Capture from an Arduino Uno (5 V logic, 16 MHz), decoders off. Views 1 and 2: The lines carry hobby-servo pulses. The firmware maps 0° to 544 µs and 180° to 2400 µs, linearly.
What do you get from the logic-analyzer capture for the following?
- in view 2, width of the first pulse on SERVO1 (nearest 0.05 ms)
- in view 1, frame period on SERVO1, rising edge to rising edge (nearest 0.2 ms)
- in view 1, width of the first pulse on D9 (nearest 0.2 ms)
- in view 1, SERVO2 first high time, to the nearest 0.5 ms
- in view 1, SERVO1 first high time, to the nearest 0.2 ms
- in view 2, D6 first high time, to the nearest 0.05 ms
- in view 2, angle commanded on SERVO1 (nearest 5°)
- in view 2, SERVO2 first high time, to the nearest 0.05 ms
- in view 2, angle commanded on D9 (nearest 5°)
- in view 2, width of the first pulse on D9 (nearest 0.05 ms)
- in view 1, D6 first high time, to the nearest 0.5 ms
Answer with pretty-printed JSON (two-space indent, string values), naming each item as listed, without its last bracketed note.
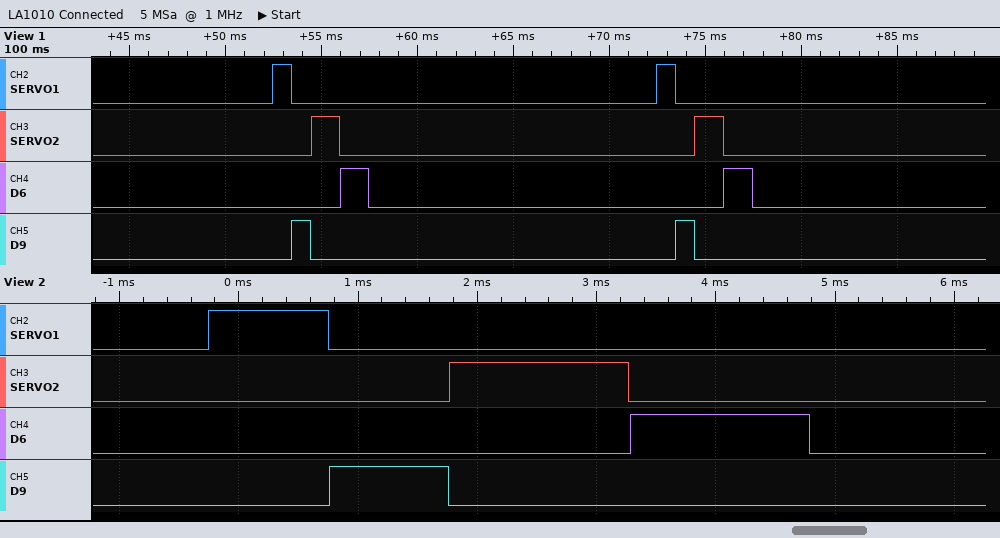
{
  "in view 2, width of the first pulse on SERVO1": "1.00 ms",
  "in view 1, frame period on SERVO1, rising edge to rising edge": "20.0 ms",
  "in view 1, width of the first pulse on D9": "1.0 ms",
  "in view 1, SERVO2 first high time, to the nearest 0.5 ms": "1.5 ms",
  "in view 1, SERVO1 first high time, to the nearest 0.2 ms": "1.0 ms",
  "in view 2, D6 first high time, to the nearest 0.05 ms": "1.50 ms",
  "in view 2, angle commanded on SERVO1": "45°",
  "in view 2, SERVO2 first high time, to the nearest 0.05 ms": "1.50 ms",
  "in view 2, angle commanded on D9": "45°",
  "in view 2, width of the first pulse on D9": "1.00 ms",
  "in view 1, D6 first high time, to the nearest 0.5 ms": "1.5 ms"
}
